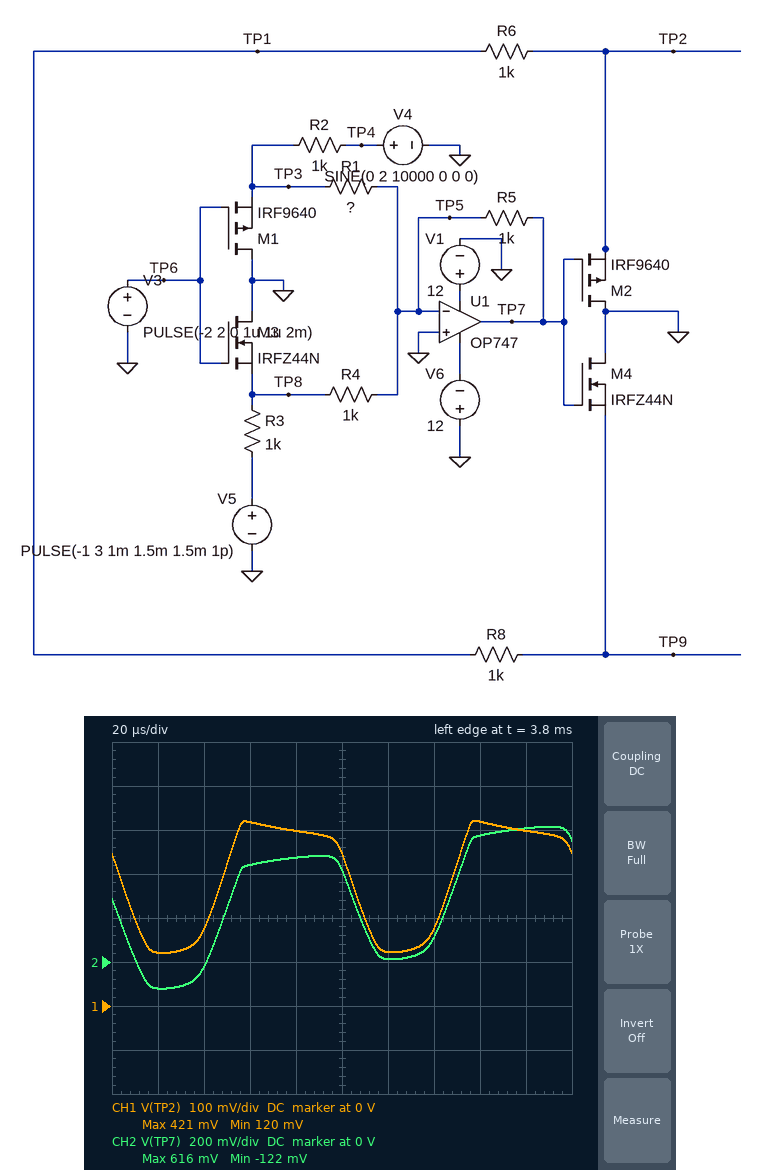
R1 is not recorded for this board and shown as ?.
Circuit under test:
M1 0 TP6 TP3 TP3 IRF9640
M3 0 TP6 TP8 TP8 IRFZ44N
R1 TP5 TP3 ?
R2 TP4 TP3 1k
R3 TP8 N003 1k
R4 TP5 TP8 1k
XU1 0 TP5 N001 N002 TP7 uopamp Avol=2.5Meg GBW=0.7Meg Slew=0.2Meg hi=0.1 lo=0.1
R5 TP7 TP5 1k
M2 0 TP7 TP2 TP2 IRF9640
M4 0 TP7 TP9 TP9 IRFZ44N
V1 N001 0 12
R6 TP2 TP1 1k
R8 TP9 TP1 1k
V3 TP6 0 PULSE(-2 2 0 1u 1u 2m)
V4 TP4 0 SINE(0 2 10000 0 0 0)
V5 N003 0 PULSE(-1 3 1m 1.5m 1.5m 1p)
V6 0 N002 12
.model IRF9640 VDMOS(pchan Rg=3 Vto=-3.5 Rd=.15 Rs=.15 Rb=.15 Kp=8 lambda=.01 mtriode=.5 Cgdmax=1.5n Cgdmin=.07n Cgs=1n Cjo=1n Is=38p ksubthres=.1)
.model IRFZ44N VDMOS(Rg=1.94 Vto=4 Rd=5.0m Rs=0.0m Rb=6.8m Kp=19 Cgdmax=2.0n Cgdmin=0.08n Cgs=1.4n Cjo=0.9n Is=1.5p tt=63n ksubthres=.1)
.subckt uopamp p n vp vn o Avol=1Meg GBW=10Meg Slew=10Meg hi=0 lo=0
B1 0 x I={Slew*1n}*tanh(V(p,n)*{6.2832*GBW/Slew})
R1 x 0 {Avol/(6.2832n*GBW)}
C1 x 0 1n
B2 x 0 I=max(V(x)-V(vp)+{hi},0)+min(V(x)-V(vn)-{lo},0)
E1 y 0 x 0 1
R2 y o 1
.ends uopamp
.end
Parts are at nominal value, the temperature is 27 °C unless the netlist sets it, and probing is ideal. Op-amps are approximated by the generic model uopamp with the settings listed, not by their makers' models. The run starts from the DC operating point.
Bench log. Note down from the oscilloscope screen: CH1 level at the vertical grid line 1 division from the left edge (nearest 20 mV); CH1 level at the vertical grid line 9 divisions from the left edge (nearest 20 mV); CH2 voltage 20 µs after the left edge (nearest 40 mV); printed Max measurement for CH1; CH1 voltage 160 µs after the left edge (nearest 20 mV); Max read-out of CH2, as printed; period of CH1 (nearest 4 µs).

120 mV
400 mV
-120 mV
421 mV
420 mV
616 mV
100 µs
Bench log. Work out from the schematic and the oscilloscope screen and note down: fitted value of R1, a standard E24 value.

3.3 kΩ
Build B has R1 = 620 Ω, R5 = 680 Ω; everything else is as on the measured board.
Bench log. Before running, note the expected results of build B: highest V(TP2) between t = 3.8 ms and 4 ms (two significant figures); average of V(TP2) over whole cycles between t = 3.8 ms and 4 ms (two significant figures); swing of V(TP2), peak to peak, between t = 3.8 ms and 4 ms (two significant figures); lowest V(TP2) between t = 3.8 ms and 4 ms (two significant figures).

420 mV
110 mV
730 mV
-310 mV
